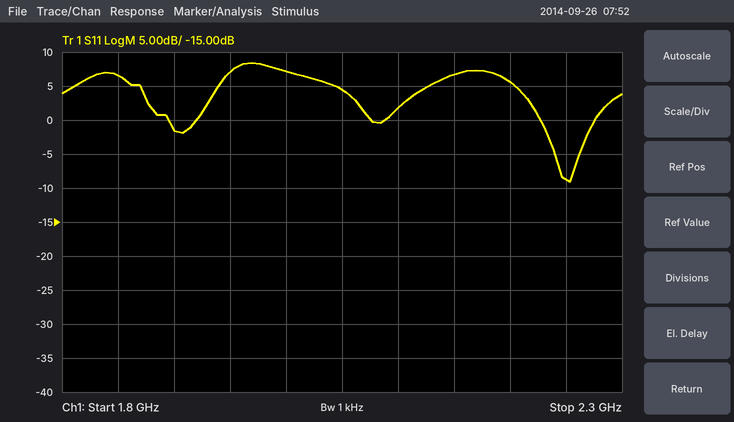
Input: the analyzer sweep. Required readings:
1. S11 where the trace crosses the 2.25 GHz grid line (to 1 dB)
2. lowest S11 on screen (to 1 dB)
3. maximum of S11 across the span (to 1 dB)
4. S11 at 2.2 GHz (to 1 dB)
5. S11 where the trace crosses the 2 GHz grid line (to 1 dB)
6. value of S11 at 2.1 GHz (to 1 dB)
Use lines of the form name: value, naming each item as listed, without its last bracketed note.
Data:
S11 where the trace crosses the 2.25 GHz grid line: -9 dB
lowest S11 on screen: -9 dB
maximum of S11 across the span: 8 dB
S11 at 2.2 GHz: 6 dB
S11 where the trace crosses the 2 GHz grid line: 7 dB
value of S11 at 2.1 GHz: 2 dB
